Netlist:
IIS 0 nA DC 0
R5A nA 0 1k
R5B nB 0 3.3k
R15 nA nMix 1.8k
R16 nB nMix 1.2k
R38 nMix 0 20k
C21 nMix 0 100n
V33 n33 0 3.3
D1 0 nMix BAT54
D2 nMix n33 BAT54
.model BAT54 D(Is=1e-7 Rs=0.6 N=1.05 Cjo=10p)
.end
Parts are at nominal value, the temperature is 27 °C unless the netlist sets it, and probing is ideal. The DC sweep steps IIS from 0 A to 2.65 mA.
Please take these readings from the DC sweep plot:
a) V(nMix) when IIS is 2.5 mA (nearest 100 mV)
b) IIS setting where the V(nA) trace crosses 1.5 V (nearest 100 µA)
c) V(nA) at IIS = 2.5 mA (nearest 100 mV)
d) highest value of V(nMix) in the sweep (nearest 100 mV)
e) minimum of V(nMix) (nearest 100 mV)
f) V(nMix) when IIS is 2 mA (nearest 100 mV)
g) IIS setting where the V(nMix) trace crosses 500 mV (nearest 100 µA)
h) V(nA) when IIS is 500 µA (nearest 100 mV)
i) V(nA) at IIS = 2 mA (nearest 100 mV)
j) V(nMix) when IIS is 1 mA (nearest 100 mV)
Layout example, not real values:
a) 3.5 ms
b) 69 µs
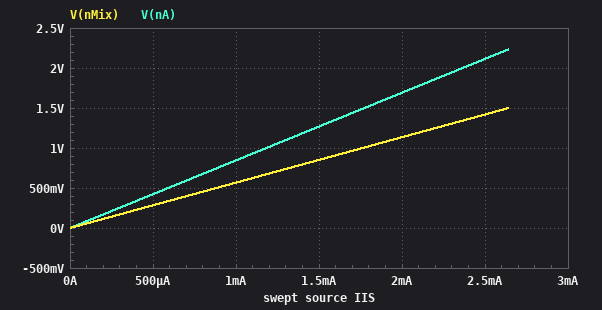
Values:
a) 1.4 V
b) 1.8 mA
c) 2.1 V
d) 1.5 V
e) 0 V
f) 1.1 V
g) 900 µA
h) 400 mV
i) 1.7 V
j) 600 mV
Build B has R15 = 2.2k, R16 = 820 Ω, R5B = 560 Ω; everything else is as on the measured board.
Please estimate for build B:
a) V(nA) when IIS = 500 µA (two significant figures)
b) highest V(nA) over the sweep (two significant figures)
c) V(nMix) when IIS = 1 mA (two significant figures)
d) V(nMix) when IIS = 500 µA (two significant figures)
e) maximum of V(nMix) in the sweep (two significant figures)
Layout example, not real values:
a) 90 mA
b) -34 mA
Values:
a) 390 mV
b) 2.1 V
c) 290 mV
d) 140 mV
e) 760 mV
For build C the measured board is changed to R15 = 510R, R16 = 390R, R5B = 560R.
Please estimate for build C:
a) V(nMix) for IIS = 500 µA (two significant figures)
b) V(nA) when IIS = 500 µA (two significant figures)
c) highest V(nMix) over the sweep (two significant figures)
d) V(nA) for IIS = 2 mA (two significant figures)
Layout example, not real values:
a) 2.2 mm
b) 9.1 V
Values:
a) 190 mV
b) 290 mV
c) 990 mV
d) 1.2 V
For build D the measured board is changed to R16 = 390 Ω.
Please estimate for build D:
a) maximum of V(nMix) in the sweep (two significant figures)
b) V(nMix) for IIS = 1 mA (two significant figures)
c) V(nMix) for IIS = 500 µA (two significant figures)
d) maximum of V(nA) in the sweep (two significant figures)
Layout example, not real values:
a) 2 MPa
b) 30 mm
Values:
a) 1.4 V
b) 530 mV
c) 260 mV
d) 2.2 V
